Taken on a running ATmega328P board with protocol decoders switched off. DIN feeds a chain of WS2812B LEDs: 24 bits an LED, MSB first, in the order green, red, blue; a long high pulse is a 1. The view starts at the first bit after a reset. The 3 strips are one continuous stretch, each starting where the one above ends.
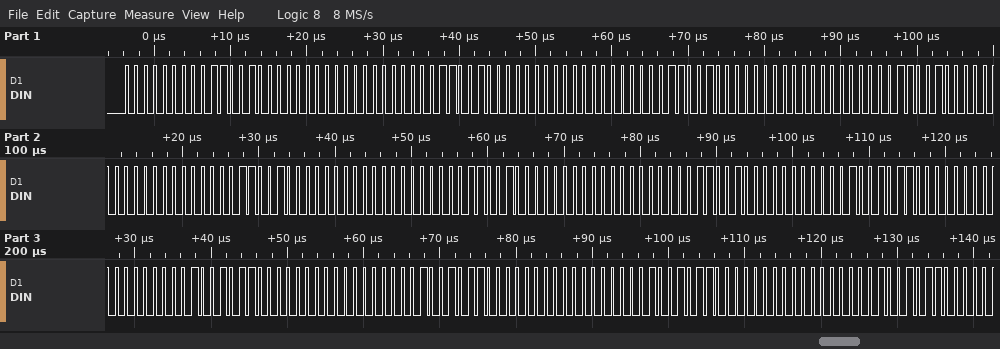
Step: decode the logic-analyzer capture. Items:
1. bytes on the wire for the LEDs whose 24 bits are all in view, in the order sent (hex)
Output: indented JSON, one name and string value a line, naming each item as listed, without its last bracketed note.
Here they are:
{
  "bytes on the wire for the LEDs whose 24 bits are all in view, in the order sent": "00 64 00 00 64 00 00 64 00 00 64 00 00 64 00 00 64 00 00 64 00 4B 00 00 4B 00 00 4B 00 00 4B 00 00"
}
